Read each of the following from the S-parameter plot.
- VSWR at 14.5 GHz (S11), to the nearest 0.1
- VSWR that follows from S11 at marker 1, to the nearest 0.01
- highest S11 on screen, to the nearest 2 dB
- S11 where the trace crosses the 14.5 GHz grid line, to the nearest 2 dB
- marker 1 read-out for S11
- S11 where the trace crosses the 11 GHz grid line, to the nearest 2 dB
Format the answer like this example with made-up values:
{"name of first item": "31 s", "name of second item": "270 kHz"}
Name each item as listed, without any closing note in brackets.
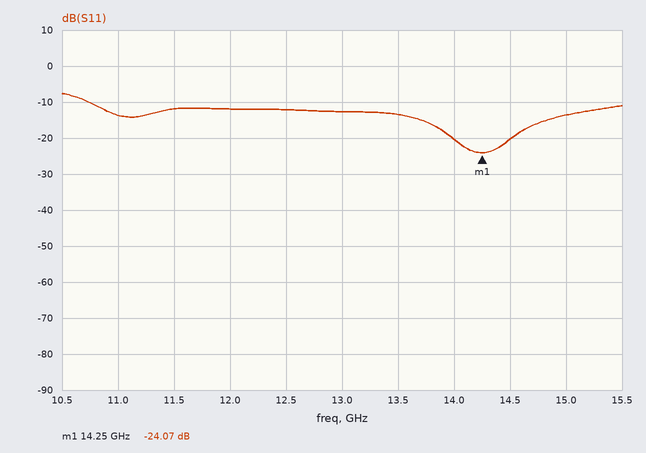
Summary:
{"VSWR at 14.5 GHz (S11), to the nearest 0.1": "1.2", "VSWR that follows from S11 at marker 1, to the nearest 0.01": "1.13", "highest S11 on screen, to the nearest 2 dB": "-8 dB", "S11 where the trace crosses the 14.5 GHz grid line, to the nearest 2 dB": "-20 dB", "marker 1 read-out for S11": "-24.07 dB", "S11 where the trace crosses the 11 GHz grid line, to the nearest 2 dB": "-14 dB"}
